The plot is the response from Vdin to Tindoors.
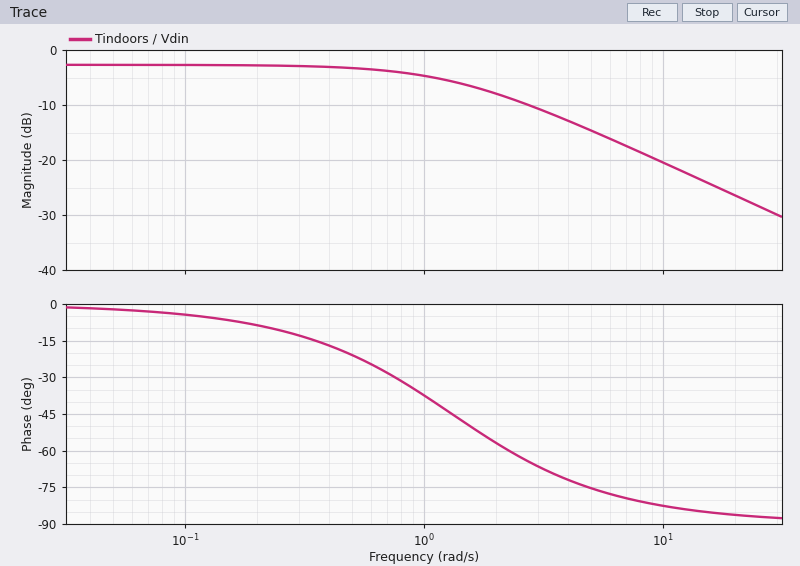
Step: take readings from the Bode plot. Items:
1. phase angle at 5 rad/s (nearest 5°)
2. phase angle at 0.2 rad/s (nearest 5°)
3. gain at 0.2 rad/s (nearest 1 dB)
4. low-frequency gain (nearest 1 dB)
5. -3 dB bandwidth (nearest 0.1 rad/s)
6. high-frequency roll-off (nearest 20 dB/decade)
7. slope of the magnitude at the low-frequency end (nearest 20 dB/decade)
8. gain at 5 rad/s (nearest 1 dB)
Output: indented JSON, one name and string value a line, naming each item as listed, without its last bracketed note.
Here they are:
{
  "phase angle at 5 rad/s": "-75°",
  "phase angle at 0.2 rad/s": "-10°",
  "gain at 0.2 rad/s": "-3 dB",
  "low-frequency gain": "-3 dB",
  "-3 dB bandwidth": "1.3 rad/s",
  "high-frequency roll-off": "-20 dB/decade",
  "slope of the magnitude at the low-frequency end": "0 dB/decade",
  "gain at 5 rad/s": "-15 dB"
}
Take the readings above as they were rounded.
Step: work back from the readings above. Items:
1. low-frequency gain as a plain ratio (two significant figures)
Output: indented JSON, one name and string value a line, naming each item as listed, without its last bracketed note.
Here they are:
{
  "low-frequency gain as a plain ratio": "0.71"
}
